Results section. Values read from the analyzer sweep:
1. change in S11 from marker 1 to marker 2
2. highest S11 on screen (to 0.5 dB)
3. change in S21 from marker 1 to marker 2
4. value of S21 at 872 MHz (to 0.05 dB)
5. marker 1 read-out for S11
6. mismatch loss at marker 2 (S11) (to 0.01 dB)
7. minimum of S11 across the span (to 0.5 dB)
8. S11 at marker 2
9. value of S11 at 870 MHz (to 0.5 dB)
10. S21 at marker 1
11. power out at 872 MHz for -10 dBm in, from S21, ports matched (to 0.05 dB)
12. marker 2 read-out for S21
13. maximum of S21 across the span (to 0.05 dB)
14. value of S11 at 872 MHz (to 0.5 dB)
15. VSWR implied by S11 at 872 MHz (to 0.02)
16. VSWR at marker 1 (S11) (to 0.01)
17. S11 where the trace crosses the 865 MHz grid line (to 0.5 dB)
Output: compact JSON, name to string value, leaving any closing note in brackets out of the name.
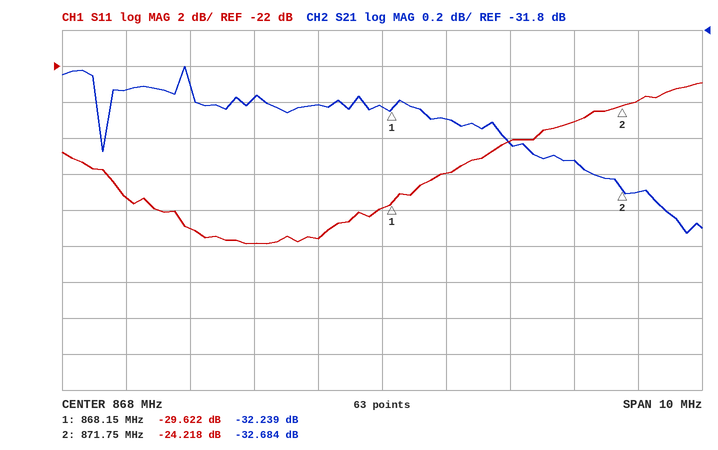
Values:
{"change in S11 from marker 1 to marker 2": "5.404 dB", "highest S11 on screen": "-23.0 dB", "change in S21 from marker 1 to marker 2": "-0.445 dB", "value of S21 at 872 MHz": "-32.70 dB", "marker 1 read-out for S11": "-29.622 dB", "mismatch loss at marker 2 (S11)": "0.02 dB", "minimum of S11 across the span": "-32.0 dB", "S11 at marker 2": "-24.218 dB", "value of S11 at 870 MHz": "-26.0 dB", "S21 at marker 1": "-32.239 dB", "power out at 872 MHz for -10 dBm in, from S21, ports matched": "-42.70 dBm", "marker 2 read-out for S21": "-32.684 dB", "maximum of S21 across the span": "-32.00 dB", "value of S11 at 872 MHz": "-24.0 dB", "VSWR implied by S11 at 872 MHz": "1.14", "VSWR at marker 1 (S11)": "1.07", "S11 where the trace crosses the 865 MHz grid line": "-31.0 dB"}
